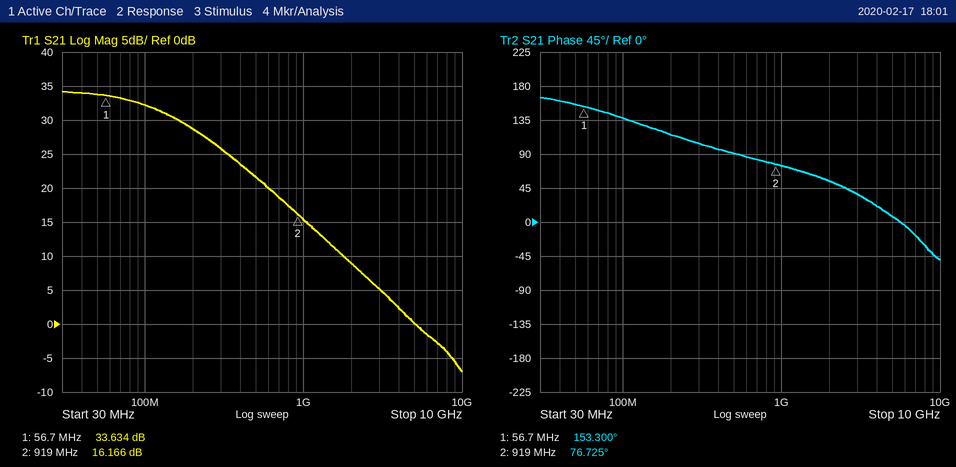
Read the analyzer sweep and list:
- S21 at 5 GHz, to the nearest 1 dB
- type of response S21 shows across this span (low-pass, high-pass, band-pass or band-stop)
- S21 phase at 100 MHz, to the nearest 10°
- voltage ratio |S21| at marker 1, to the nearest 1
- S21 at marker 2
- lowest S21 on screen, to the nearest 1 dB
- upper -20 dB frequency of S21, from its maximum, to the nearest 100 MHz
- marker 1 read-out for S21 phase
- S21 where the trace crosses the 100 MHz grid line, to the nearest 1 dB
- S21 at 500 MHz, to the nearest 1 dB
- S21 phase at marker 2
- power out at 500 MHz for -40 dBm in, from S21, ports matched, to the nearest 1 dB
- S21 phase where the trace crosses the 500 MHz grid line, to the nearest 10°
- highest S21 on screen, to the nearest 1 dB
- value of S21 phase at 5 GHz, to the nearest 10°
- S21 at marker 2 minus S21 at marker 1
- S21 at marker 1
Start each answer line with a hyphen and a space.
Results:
- 0 dB
- low-pass
- 140°
- 48
- 16.166 dB
- -7 dB
- 1.1 GHz
- 153.300°
- 32 dB
- 22 dB
- 76.725°
- -18 dBm
- 90°
- 34 dB
- 10°
- -17.468 dB
- 33.634 dB
